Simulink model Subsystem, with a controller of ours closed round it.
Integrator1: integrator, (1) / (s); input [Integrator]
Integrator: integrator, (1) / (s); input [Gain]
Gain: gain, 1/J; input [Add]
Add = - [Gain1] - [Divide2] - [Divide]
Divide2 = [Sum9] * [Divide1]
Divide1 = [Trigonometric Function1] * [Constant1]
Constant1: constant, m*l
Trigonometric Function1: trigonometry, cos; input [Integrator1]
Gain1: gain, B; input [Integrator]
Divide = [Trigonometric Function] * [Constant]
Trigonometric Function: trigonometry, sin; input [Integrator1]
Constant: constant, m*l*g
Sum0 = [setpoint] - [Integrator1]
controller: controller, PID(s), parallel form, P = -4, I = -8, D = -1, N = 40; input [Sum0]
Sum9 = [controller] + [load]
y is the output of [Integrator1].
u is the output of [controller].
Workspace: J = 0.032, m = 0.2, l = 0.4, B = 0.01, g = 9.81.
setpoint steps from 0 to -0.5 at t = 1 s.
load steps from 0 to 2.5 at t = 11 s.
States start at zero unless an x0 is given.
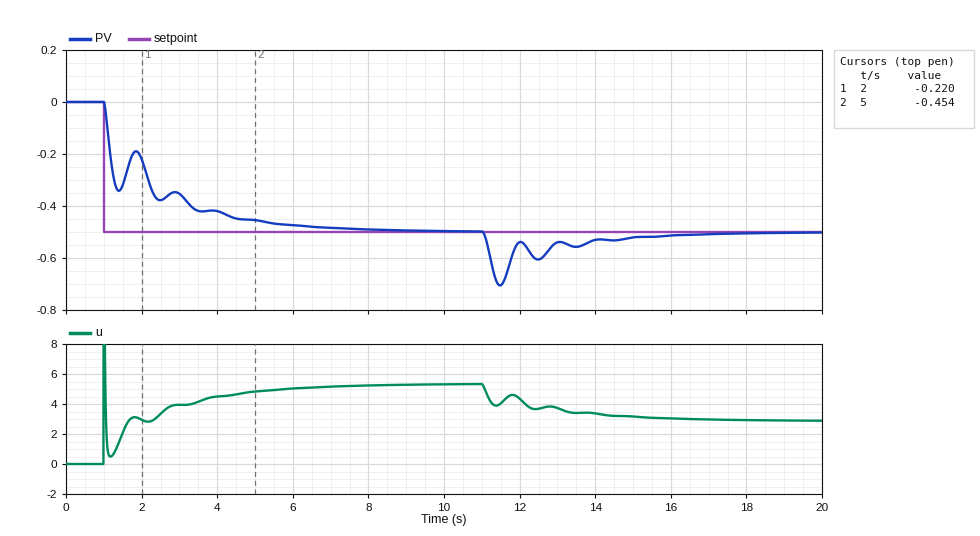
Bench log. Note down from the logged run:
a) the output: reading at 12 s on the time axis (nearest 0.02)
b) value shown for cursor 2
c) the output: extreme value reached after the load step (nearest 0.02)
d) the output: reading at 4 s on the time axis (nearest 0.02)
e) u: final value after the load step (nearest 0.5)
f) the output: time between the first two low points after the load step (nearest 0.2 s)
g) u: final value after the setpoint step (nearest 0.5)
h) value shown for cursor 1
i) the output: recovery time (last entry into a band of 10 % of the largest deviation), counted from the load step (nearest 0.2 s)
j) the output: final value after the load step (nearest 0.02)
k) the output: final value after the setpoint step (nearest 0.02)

-0.54
-0.454
-0.70
-0.42
3.0
1.0 s
5.5
-0.220
4.0 s
-0.50
-0.50
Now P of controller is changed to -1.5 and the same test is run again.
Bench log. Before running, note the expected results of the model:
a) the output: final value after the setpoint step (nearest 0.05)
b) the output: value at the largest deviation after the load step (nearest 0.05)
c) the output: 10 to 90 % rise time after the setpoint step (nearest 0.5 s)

-0.50
-0.75
3.5 s
